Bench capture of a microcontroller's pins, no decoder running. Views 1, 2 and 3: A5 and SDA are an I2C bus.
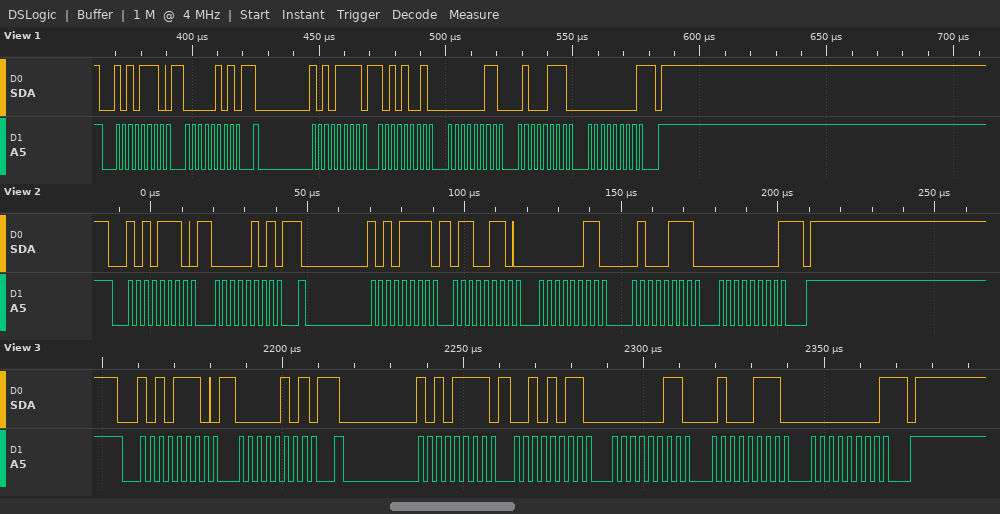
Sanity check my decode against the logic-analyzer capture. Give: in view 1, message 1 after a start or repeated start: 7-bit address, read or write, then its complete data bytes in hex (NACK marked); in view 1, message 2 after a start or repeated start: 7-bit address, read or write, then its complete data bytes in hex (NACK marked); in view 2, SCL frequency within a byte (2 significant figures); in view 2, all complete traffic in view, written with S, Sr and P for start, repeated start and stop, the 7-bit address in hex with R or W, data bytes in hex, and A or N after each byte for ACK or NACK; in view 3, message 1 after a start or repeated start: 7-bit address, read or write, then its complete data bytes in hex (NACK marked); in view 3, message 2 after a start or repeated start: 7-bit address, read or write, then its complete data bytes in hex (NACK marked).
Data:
0x57 write: 05
0x57 read: A9 03 47 00 NACK
400 kHz
S 57W A 05 A Sr 57R A 66 A 03 A 47 A 00 N P
0x57 write: 05
0x57 read: 2B 03 47 00 NACK
